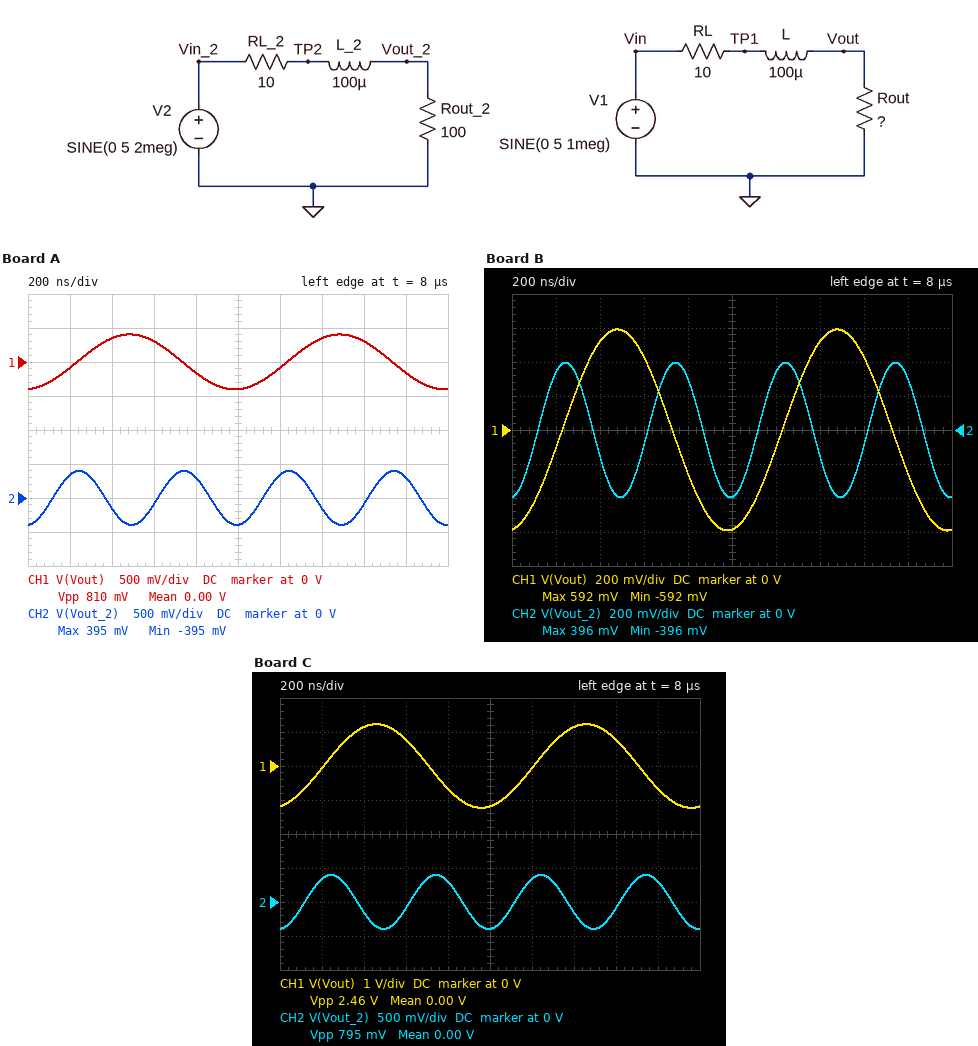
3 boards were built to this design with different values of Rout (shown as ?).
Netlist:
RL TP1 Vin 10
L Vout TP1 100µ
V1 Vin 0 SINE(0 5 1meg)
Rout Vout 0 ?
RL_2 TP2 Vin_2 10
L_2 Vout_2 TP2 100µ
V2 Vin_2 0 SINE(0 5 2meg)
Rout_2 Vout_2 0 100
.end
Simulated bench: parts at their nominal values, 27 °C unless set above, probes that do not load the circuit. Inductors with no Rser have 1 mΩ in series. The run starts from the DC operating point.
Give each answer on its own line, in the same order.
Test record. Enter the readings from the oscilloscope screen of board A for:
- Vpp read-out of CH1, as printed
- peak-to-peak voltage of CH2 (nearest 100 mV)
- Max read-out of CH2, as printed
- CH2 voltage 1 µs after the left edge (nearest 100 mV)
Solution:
810 mV
800 mV
395 mV
-400 mV
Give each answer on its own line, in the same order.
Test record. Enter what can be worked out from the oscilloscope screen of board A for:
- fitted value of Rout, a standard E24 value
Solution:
51 Ω
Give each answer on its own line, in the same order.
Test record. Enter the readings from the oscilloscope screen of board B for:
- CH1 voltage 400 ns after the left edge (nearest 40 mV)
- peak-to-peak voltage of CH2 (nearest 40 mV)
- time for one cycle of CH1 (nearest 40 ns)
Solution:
520 mV
800 mV
1.00 µs
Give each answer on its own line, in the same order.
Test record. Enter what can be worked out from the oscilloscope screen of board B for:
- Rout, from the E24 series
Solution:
75 Ω
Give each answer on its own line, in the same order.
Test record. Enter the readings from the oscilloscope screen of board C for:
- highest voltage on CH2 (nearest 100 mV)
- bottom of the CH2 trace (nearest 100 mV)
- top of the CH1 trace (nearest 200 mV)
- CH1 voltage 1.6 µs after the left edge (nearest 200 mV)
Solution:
400 mV
-400 mV
1.2 V
800 mV
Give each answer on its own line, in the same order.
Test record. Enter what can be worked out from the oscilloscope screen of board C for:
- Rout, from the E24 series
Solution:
160 Ω
